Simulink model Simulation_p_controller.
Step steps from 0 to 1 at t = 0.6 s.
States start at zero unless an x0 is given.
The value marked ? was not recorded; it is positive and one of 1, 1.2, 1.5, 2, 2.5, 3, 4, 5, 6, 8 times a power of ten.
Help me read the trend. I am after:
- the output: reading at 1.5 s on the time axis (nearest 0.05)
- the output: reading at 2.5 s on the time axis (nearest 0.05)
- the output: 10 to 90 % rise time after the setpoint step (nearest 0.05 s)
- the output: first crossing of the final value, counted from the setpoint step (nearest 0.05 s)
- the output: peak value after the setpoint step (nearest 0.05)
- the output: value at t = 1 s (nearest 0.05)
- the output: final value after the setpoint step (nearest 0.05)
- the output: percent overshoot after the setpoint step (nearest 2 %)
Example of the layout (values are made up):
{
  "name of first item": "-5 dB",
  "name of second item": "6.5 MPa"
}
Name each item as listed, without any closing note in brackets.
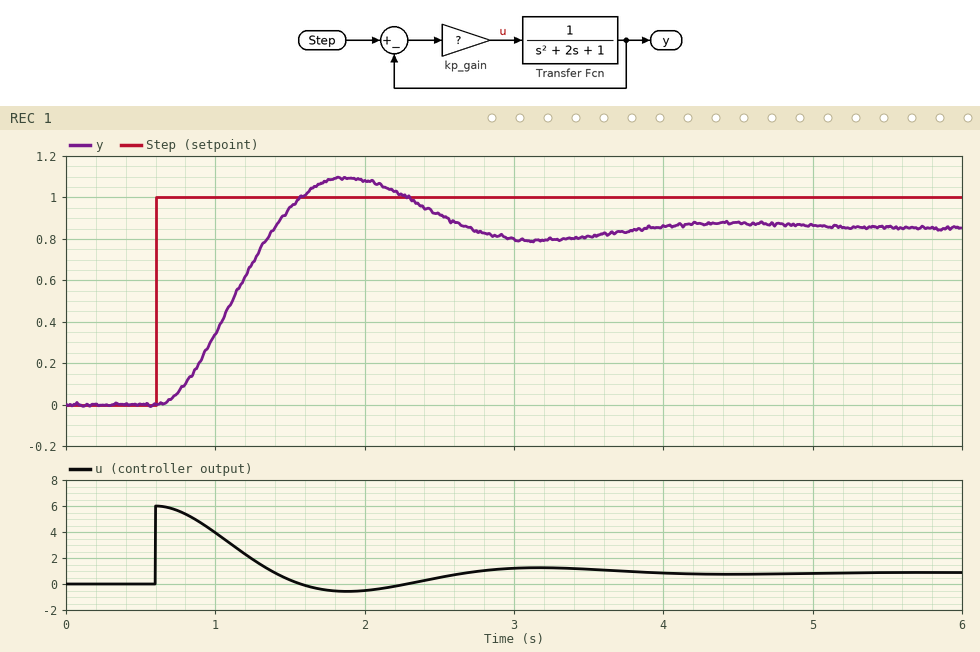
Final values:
{
  "the output: reading at 1.5 s on the time axis": "0.95",
  "the output: reading at 2.5 s on the time axis": "0.90",
  "the output: 10 to 90 % rise time after the setpoint step": "0.55 s",
  "the output: first crossing of the final value, counted from the setpoint step": "0.80 s",
  "the output: peak value after the setpoint step": "1.10",
  "the output: value at t = 1 s": "0.35",
  "the output: final value after the setpoint step": "0.85",
  "the output: percent overshoot after the setpoint step": "28 %"
}
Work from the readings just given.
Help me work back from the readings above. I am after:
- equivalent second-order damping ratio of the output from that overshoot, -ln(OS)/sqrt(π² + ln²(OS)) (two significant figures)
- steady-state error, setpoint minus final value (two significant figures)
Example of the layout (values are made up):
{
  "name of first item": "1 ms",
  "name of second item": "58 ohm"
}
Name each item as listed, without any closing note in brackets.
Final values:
{
  "equivalent second-order damping ratio of the output from that overshoot, -ln(OS)/sqrt(π² + ln²(OS))": "0.38",
  "steady-state error, setpoint minus final value": "0.15"
}
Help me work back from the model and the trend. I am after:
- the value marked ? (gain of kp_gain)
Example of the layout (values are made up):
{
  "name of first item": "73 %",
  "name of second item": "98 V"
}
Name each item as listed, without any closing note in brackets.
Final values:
{
  "the value marked ?": "6"
}
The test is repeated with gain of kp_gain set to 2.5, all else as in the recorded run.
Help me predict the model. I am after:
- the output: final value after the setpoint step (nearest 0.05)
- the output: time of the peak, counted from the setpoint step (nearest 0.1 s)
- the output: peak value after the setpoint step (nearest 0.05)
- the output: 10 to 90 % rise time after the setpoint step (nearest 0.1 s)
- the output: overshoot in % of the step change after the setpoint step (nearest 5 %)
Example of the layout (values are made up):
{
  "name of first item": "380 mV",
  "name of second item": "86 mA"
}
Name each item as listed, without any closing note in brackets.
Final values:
{
  "the output: final value after the setpoint step": "0.70",
  "the output: time of the peak, counted from the setpoint step": "2.0 s",
  "the output: peak value after the setpoint step": "0.80",
  "the output: 10 to 90 % rise time after the setpoint step": "0.9 s",
  "the output: overshoot in % of the step change after the setpoint step": "15 %"
}
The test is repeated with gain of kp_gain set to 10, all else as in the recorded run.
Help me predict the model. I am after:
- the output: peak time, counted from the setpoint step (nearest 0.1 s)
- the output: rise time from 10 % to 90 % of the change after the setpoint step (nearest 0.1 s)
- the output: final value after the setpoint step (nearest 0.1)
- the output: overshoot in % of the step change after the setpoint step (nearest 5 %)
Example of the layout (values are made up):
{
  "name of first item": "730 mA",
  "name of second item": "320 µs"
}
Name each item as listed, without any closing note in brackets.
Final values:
{
  "the output: peak time, counted from the setpoint step": "1.0 s",
  "the output: rise time from 10 % to 90 % of the change after the setpoint step": "0.4 s",
  "the output: final value after the setpoint step": "0.9",
  "the output: overshoot in % of the step change after the setpoint step": "35 %"
}
